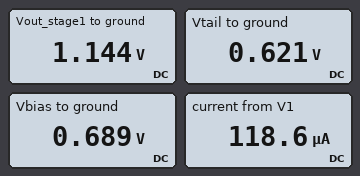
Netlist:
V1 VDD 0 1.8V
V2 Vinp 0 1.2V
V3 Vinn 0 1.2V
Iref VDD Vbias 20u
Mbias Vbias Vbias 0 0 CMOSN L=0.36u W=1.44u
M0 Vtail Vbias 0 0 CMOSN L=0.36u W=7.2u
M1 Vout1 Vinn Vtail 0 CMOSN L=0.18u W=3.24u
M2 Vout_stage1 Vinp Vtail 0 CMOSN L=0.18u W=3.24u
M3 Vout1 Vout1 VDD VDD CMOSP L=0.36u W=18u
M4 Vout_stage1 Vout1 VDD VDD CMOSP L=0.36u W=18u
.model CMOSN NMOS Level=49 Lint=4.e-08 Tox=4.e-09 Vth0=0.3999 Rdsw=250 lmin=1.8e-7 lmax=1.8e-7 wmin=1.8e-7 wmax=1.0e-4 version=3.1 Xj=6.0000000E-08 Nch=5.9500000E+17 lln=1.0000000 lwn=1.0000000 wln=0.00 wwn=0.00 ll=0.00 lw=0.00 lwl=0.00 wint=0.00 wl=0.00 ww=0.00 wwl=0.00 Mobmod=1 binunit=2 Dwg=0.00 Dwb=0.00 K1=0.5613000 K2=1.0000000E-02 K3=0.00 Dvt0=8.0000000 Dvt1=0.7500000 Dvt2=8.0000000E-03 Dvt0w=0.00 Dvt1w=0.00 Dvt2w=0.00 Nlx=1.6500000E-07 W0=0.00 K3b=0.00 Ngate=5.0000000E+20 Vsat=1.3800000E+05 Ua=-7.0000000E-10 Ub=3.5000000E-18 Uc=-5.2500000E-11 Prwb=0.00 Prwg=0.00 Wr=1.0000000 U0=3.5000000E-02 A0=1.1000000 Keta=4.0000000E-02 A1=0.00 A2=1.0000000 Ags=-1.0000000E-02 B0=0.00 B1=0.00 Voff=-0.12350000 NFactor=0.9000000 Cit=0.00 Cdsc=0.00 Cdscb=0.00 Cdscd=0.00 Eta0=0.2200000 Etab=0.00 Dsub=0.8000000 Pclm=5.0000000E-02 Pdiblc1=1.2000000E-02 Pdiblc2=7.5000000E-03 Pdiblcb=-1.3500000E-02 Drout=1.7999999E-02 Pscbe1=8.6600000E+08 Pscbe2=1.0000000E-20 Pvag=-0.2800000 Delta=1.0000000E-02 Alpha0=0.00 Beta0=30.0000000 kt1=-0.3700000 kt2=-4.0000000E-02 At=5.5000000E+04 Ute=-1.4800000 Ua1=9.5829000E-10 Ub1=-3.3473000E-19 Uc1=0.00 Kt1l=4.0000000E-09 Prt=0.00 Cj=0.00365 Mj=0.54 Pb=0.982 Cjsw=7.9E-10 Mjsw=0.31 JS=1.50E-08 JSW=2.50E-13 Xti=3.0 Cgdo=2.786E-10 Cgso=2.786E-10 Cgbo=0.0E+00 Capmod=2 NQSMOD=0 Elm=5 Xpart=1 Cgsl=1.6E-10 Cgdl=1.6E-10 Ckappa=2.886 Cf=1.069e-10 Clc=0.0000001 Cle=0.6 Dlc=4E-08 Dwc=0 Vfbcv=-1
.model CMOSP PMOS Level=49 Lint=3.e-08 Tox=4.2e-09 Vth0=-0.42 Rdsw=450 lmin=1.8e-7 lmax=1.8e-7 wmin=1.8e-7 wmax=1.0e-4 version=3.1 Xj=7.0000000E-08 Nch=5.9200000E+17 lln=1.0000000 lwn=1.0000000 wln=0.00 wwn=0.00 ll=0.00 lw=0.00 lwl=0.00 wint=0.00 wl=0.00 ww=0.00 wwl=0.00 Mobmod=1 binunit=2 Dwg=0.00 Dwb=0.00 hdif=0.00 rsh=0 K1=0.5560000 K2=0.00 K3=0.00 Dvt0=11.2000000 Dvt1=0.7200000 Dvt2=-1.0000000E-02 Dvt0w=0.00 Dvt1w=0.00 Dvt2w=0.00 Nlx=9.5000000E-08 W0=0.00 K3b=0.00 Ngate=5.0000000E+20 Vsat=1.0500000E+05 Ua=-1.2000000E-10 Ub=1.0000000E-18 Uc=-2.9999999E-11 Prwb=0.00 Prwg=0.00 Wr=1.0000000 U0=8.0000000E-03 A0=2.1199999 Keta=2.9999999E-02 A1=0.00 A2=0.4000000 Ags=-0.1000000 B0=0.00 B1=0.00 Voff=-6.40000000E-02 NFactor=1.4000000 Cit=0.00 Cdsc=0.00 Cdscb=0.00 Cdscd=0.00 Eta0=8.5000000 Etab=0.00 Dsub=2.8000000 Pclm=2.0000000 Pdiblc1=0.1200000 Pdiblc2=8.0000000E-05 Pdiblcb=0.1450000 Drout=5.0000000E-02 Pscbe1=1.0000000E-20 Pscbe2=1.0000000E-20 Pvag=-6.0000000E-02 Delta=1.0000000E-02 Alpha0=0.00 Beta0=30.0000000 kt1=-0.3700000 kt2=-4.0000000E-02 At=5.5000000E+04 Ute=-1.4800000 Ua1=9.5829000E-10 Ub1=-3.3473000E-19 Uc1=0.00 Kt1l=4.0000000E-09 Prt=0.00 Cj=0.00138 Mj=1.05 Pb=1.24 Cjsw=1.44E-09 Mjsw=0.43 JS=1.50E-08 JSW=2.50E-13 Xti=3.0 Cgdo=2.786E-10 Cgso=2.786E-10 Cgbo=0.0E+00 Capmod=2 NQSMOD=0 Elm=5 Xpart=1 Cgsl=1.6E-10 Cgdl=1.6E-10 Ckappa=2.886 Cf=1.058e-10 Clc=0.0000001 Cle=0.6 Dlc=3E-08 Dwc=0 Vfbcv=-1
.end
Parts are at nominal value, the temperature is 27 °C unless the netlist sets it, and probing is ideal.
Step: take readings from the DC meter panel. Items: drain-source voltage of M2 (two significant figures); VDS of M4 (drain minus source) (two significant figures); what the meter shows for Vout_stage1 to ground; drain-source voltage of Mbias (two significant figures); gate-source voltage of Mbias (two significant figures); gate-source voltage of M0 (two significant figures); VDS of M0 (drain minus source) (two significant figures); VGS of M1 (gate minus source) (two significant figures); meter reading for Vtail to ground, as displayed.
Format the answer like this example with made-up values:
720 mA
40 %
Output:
520 mV
-660 mV
1.144 V
690 mV
690 mV
690 mV
620 mV
580 mV
0.621 V
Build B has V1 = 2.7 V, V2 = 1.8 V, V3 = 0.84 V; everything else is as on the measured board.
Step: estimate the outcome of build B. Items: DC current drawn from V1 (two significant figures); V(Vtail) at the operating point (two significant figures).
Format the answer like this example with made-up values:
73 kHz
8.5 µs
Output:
110 µA
400 mV
